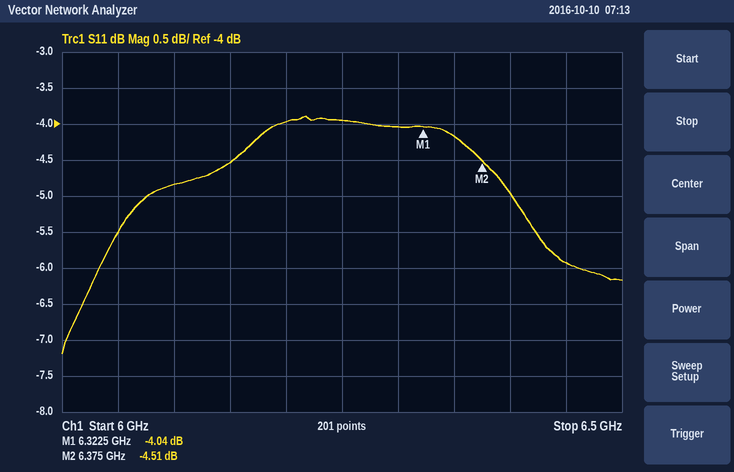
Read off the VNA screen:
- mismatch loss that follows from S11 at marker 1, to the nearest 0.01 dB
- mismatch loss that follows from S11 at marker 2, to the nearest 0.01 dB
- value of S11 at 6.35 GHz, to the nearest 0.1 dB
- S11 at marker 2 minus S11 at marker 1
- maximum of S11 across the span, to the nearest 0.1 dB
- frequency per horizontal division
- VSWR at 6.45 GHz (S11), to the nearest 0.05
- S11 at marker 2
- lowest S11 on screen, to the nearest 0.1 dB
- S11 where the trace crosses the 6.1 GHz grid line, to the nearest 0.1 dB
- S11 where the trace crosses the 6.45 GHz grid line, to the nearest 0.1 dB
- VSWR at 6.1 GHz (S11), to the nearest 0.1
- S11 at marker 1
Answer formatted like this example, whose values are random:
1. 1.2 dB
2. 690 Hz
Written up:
1. 2.18 dB
2. 1.90 dB
3. -4.2 dB
4. -0.47 dB
5. -3.9 dB
6. 50 MHz
7. 3.05
8. -4.51 dB
9. -7.2 dB
10. -4.8 dB
11. -5.9 dB
12. 3.7
13. -4.04 dB
